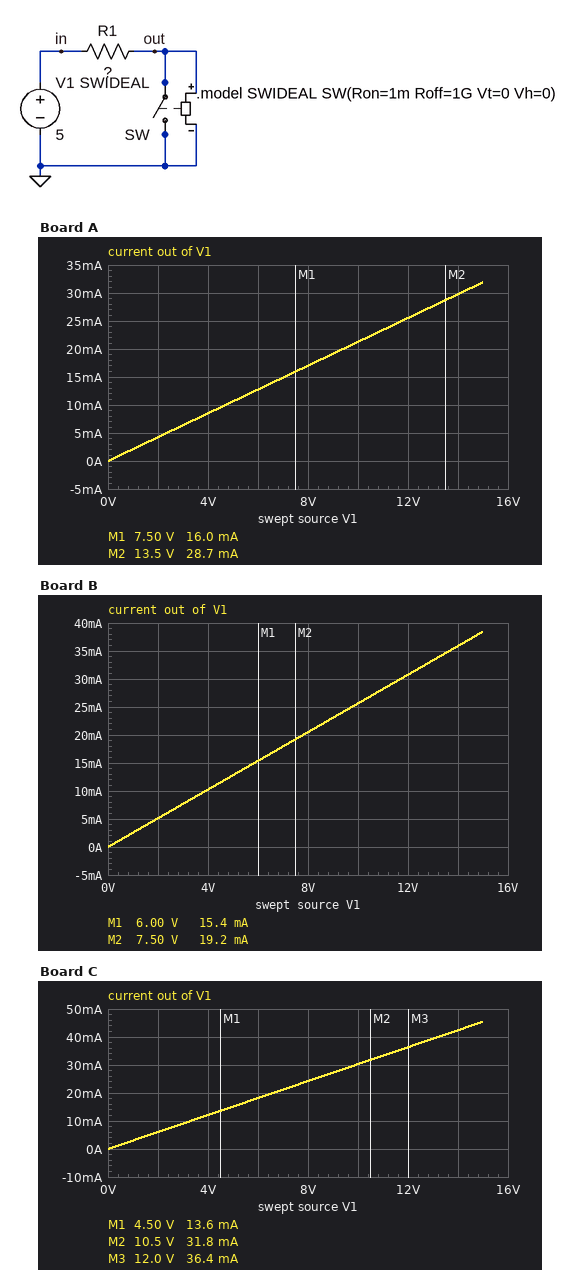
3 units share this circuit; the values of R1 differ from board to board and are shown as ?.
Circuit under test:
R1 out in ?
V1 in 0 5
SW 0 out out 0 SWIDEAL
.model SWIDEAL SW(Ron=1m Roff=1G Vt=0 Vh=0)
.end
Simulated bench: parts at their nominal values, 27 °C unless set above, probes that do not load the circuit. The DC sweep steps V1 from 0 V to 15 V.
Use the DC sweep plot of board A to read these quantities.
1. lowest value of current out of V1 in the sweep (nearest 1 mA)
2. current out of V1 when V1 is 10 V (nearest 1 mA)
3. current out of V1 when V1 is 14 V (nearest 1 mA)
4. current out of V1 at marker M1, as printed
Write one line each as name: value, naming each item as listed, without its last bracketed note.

lowest value of current out of V1 in the sweep: 0 A
current out of V1 when V1 is 10 V: 21 mA
current out of V1 when V1 is 14 V: 30 mA
current out of V1 at marker M1, as printed: 16.0 mA
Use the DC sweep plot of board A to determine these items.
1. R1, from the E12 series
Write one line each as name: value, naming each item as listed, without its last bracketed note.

R1, from the E12 series: 470 Ω
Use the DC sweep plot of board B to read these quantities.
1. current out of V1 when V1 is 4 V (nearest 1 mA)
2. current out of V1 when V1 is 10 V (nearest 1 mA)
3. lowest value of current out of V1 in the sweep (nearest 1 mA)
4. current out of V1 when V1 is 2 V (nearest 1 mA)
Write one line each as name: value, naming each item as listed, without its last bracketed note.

current out of V1 when V1 is 4 V: 10 mA
current out of V1 when V1 is 10 V: 26 mA
lowest value of current out of V1 in the sweep: 0 A
current out of V1 when V1 is 2 V: 5 mA
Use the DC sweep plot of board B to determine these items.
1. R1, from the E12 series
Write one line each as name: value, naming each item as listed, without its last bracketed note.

R1, from the E12 series: 390 Ω
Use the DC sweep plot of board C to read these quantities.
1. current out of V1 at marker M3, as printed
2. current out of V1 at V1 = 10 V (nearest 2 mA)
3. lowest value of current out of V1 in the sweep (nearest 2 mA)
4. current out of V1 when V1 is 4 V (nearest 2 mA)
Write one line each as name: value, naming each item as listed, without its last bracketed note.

current out of V1 at marker M3, as printed: 36.4 mA
current out of V1 at V1 = 10 V: 30 mA
lowest value of current out of V1 in the sweep: 0 A
current out of V1 when V1 is 4 V: 12 mA
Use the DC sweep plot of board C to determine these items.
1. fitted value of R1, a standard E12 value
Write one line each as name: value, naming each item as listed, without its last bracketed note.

fitted value of R1, a standard E12 value: 330 Ω
